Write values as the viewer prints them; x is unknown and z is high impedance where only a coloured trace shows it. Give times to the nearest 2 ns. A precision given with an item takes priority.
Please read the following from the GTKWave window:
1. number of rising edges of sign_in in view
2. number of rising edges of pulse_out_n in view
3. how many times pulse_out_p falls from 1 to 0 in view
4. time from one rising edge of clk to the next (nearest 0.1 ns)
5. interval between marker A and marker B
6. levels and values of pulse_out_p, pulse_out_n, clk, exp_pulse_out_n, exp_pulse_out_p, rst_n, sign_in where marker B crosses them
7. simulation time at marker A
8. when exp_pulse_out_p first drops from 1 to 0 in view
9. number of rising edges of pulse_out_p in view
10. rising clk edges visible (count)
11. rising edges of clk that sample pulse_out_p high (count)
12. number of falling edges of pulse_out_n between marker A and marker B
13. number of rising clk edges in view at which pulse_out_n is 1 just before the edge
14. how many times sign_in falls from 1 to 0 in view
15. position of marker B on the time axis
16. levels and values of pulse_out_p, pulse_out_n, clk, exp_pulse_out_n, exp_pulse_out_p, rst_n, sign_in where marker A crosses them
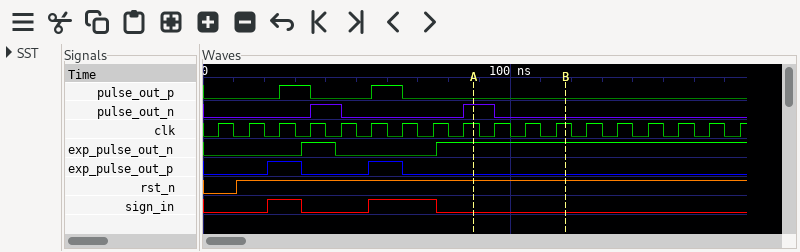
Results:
2
2
2
10 ns
30 ns
pulse_out_p=0, pulse_out_n=0, clk=1, exp_pulse_out_n=1, exp_pulse_out_p=0, rst_n=1, sign_in=0
88 ns
32 ns
2
18
2
1
2
2
118 ns
pulse_out_p=0, pulse_out_n=1, clk=1, exp_pulse_out_n=1, exp_pulse_out_p=0, rst_n=1, sign_in=0
